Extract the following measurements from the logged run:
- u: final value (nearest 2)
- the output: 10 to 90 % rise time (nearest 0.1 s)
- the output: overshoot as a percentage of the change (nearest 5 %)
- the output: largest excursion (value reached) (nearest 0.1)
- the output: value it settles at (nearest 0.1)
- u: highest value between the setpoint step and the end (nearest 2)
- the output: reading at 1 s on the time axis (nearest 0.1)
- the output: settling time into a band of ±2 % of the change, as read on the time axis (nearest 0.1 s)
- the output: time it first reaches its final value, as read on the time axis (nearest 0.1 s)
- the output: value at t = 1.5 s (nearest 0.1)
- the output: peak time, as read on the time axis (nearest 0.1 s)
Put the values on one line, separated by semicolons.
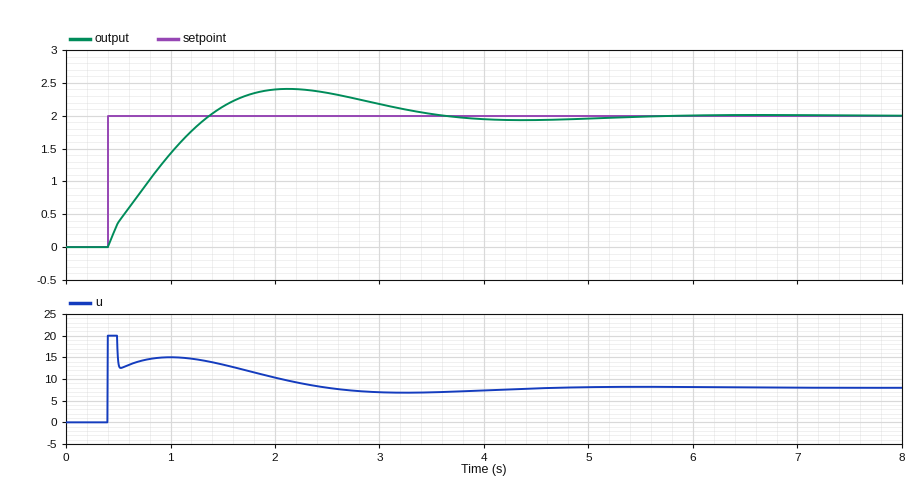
8; 0.8 s; 20 %; 2.4; 2.0; 20; 1.4; 5.1 s; 1.4 s; 2.1; 2.1 s
